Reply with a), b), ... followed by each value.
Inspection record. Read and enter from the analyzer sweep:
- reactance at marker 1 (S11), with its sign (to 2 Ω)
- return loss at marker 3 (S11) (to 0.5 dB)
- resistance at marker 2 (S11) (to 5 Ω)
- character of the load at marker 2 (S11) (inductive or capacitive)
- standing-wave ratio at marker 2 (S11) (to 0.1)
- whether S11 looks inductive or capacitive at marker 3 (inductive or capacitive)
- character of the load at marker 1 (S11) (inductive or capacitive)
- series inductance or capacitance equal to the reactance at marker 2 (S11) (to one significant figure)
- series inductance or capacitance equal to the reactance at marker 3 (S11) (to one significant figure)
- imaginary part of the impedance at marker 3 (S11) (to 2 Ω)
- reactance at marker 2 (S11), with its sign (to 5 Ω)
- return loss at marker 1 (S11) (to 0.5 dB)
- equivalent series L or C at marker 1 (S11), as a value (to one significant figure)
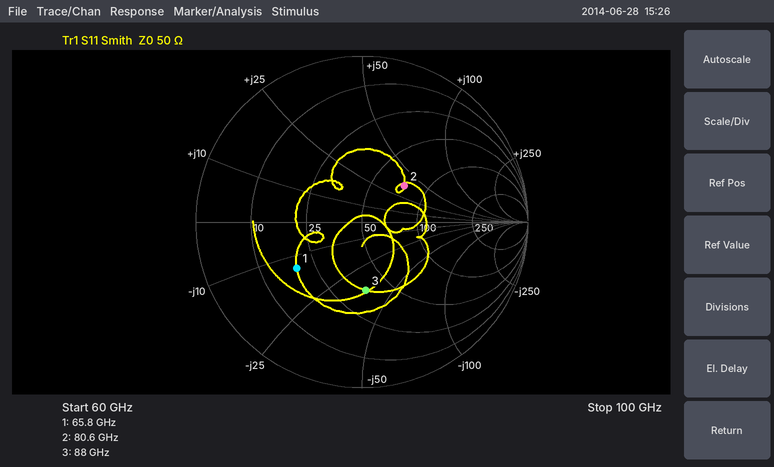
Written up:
a) -14 Ω
b) 7.5 dB
c) 75 Ω
d) inductive
e) 2.0
f) capacitive
g) capacitive
h) 70 pH
i) 50 fF
j) -36 Ω
k) +35 Ω
l) 6.5 dB
m) 200 fF
